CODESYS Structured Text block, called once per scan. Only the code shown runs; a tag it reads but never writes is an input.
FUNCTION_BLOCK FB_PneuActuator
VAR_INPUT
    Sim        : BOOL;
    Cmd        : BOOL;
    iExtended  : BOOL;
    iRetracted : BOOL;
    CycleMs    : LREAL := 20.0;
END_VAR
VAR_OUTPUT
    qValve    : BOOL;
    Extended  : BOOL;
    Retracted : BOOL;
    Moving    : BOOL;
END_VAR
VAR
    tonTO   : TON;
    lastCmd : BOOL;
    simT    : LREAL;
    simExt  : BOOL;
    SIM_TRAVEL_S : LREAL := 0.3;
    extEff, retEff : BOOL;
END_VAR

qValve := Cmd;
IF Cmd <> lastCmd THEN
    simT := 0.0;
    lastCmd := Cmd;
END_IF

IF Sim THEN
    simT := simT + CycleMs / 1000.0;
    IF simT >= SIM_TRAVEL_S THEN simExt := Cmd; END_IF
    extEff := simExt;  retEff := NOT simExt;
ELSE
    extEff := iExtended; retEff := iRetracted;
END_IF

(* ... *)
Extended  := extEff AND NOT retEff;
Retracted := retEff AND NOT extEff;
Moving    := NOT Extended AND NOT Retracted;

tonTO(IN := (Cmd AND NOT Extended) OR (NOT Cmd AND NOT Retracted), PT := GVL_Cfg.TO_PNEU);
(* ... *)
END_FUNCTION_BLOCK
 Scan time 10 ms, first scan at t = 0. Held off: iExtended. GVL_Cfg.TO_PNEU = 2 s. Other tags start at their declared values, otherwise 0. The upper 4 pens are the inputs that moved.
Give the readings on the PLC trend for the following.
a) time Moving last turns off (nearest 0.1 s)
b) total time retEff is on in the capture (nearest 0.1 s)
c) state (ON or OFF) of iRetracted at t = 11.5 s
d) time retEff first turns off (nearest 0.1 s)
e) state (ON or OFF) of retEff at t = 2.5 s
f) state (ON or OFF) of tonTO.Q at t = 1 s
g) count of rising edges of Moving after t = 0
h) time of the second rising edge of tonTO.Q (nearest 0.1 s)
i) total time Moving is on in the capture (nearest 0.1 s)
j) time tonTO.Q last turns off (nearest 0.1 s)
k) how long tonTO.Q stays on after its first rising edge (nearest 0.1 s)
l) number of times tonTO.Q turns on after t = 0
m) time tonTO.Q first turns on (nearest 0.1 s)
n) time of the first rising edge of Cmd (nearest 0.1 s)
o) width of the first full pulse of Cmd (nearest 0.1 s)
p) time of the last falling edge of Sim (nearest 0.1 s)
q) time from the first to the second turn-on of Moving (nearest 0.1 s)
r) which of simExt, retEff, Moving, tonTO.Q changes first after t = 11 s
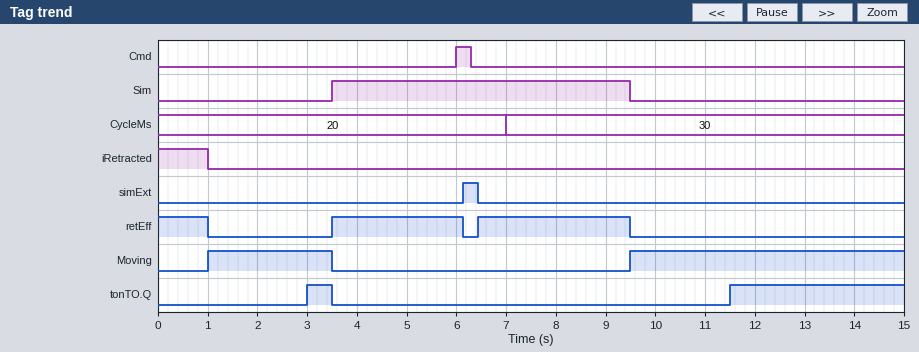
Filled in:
3.5 s
6.7 s
OFF
1.0 s
OFF
OFF
2
11.5 s
8.0 s
3.5 s
0.5 s
2
3.0 s
6.0 s
0.3 s
9.5 s
8.5 s
tonTO.Q
